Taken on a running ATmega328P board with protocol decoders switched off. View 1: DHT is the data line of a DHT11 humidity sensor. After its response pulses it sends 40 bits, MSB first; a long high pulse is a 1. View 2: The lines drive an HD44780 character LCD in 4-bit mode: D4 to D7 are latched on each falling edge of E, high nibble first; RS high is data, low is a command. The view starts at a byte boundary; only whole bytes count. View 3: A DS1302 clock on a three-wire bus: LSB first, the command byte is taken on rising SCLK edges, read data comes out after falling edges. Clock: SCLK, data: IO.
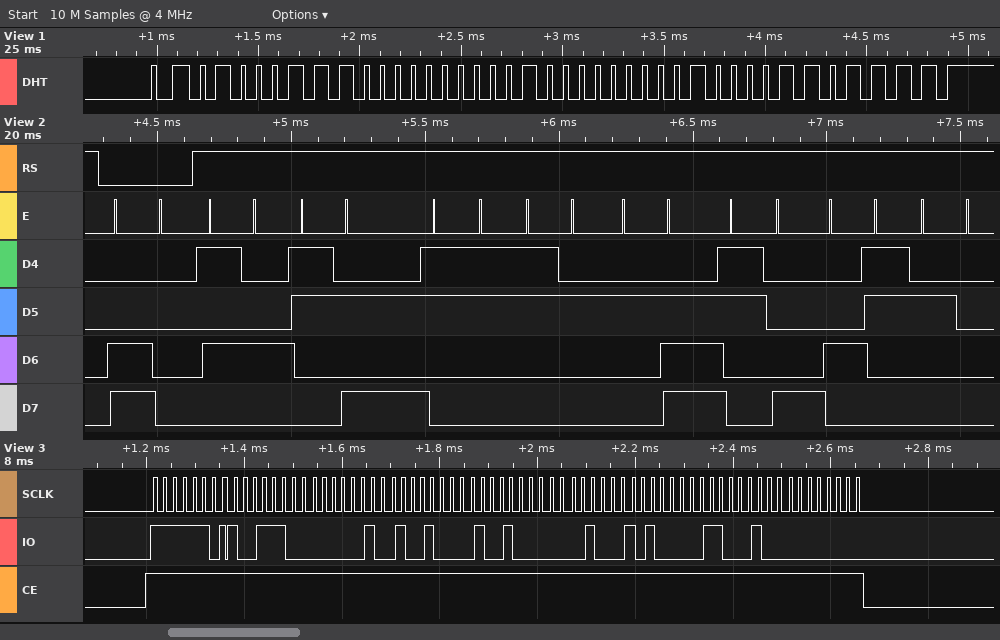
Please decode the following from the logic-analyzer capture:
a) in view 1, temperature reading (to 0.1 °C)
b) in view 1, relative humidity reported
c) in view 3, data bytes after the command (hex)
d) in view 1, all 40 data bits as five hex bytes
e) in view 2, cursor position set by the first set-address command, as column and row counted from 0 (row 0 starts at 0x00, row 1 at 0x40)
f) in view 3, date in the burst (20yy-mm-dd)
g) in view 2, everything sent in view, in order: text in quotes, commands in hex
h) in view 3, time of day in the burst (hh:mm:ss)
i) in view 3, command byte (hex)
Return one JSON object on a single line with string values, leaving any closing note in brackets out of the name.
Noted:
{"in view 1, temperature reading": "32.8 °C", "in view 1, relative humidity reported": "71 %", "in view 3, data bytes after the command": "39 40 12 12 10 05 23 00", "in view 1, all 40 data bits as five hex bytes": "47 00 20 08 6F", "in view 2, cursor position set by the first set-address command, as column and row counted from 0": "column 0, row 1", "in view 3, date in the burst": "2023-10-12", "in view 2, everything sent in view, in order: text in quotes, commands in hex": "0xC0 \"T:32.8C \"", "in view 3, time of day in the burst": "12:40:39", "in view 3, command byte": "0xBF"}
